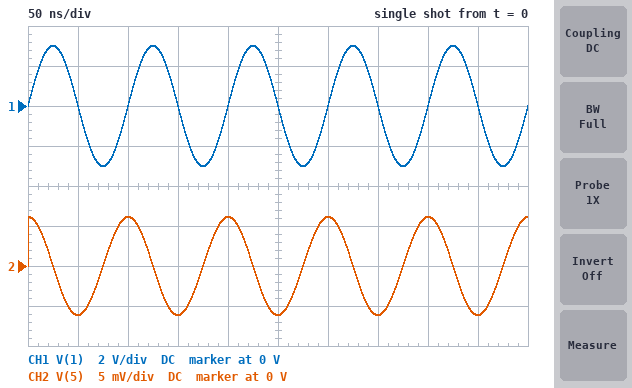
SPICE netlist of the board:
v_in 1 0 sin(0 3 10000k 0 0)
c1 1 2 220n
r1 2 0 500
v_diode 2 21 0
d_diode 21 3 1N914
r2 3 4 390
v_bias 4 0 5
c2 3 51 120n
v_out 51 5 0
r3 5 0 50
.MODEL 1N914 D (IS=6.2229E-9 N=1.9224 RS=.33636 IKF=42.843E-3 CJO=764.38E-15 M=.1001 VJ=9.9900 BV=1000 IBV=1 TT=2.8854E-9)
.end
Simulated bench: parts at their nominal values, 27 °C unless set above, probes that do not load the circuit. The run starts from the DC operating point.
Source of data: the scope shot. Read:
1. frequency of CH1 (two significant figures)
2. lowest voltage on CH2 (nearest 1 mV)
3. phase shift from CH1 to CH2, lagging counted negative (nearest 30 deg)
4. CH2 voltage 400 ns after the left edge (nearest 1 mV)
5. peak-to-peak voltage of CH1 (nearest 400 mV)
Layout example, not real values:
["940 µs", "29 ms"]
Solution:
["10 MHz", "-6 mV", "90 deg", "6 mV", "6.0 V"]
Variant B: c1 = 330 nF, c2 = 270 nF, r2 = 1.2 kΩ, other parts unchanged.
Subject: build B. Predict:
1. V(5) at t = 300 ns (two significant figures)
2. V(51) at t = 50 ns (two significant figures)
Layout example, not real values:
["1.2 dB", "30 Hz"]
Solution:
["6.6 mV", "-6.6 mV"]
